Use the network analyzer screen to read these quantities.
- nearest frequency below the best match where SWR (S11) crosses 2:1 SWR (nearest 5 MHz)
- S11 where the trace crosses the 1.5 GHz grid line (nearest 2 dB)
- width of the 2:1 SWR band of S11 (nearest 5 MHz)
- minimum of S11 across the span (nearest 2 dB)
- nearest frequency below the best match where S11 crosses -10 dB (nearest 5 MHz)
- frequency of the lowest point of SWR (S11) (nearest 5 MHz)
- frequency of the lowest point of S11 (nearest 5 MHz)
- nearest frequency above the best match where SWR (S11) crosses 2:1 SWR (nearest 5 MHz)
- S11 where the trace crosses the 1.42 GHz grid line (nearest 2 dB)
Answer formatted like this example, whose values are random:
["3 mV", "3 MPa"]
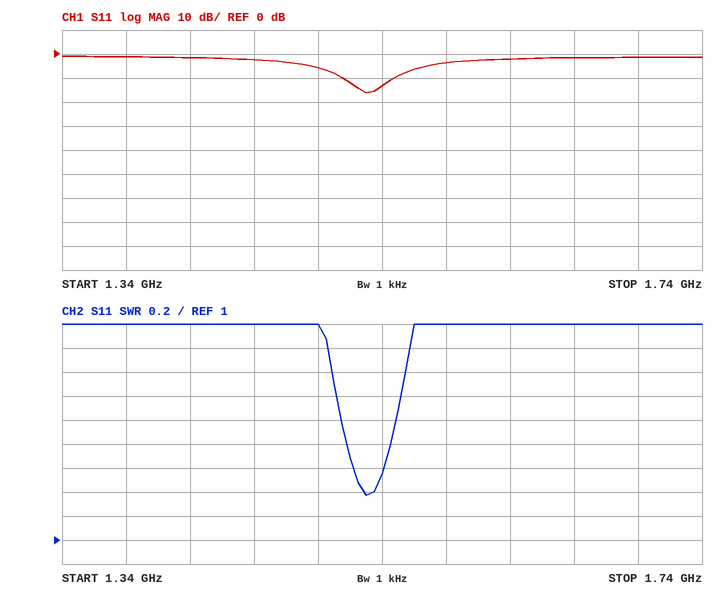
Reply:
["1.515 GHz", "-6 dB", "35 MHz", "-16 dB", "1.515 GHz", "1.530 GHz", "1.530 GHz", "1.550 GHz", "-2 dB"]
